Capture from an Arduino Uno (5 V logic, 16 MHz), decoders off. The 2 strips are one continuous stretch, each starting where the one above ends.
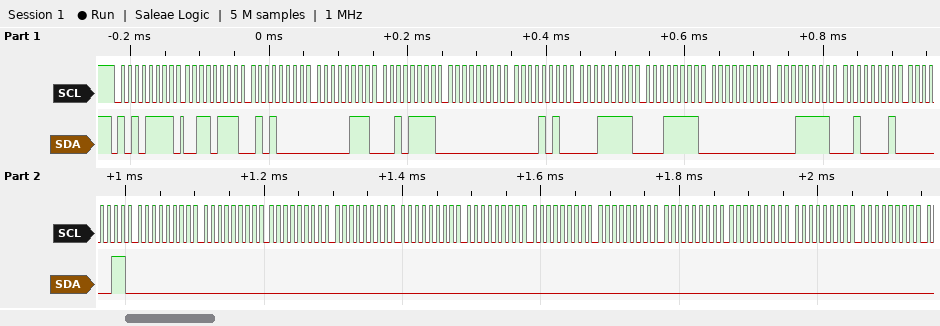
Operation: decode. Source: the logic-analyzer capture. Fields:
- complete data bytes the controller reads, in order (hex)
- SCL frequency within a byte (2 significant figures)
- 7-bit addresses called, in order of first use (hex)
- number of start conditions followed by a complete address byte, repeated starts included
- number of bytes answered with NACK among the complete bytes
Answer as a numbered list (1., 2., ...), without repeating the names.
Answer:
1. 37 50 07 2F 00 0A 1F 1F 00 1F 21 03 00 00 00 00 00 00 00 00 00 00 00 00
2. 100 kHz
3. 0x57
4. 1
5. 0
